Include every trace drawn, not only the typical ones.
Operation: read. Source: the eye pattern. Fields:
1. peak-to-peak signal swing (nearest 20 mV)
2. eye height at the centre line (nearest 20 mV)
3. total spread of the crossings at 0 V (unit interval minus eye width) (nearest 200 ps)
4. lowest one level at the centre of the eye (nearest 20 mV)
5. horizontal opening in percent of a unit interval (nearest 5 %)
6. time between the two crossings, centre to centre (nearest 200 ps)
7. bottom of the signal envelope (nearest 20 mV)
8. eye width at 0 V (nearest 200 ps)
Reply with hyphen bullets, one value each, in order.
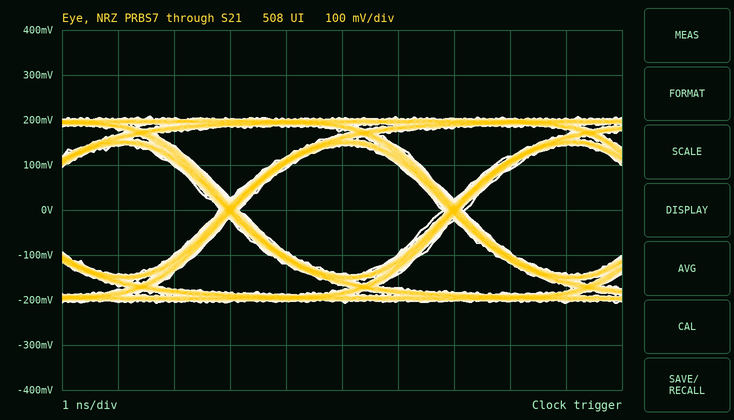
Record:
- 420 mV
- 280 mV
- 400 ps
- 140 mV
- 90 %
- 4.0 ns
- -200 mV
- 3.6 ns
